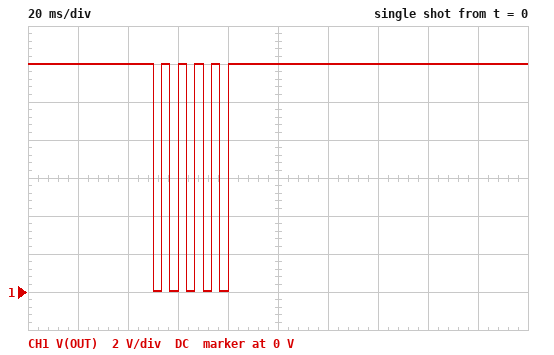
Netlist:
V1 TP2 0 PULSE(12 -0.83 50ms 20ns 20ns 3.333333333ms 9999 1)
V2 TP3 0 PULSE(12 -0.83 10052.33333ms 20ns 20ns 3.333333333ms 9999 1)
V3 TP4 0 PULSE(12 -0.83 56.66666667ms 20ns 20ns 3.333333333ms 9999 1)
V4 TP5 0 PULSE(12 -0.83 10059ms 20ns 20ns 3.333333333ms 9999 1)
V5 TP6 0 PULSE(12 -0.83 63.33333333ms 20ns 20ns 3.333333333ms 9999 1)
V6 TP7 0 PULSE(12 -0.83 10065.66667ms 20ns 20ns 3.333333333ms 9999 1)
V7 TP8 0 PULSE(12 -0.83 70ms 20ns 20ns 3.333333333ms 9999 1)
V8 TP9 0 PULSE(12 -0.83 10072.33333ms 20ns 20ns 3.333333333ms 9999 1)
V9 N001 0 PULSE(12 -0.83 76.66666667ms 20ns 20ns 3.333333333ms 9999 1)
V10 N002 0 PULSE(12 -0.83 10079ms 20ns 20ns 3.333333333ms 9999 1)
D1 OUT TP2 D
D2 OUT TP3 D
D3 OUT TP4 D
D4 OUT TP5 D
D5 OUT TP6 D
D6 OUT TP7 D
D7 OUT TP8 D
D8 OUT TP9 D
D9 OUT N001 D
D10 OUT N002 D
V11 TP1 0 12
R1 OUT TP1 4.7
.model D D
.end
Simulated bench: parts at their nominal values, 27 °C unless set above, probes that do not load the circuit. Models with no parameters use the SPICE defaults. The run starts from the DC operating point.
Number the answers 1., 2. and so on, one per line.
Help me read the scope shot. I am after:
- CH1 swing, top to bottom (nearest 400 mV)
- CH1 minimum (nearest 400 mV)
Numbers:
1. 12.0 V
2. 0 V
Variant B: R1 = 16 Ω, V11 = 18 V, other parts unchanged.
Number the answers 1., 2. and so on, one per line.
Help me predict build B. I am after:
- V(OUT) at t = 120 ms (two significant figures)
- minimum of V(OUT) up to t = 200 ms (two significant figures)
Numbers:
1. 13 V
2. 6.8 mV
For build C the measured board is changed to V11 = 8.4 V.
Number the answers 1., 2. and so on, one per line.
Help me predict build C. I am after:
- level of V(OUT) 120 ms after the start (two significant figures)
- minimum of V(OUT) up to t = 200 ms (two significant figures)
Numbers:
1. 8.4 V
2. 19 mV
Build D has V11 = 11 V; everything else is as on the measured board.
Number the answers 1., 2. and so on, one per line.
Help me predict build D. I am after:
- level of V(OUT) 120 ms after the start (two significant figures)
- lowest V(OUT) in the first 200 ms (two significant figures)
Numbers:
1. 11 V
2. 26 mV
